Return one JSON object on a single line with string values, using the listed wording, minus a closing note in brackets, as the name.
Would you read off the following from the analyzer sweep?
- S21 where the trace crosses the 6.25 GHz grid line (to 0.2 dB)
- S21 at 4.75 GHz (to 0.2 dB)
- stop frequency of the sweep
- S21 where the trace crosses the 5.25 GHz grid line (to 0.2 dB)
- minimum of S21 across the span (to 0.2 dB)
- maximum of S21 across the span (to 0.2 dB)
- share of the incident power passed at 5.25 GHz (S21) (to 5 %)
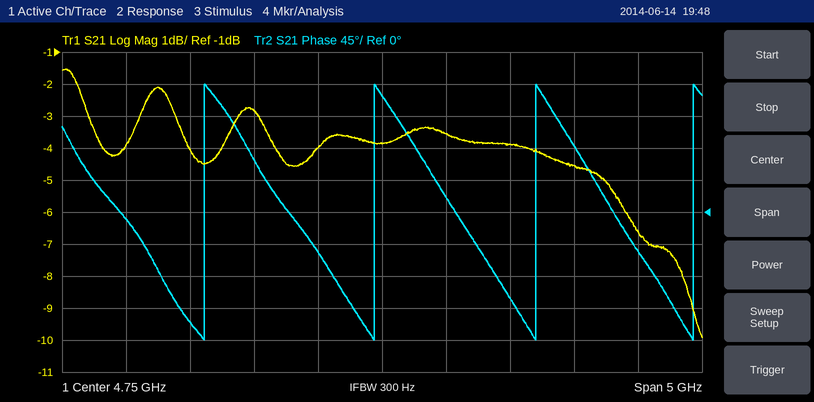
{"S21 where the trace crosses the 6.25 GHz grid line": "-4.6 dB", "S21 at 4.75 GHz": "-3.8 dB", "stop frequency of the sweep": "7.25 GHz", "S21 where the trace crosses the 5.25 GHz grid line": "-3.6 dB", "minimum of S21 across the span": "-10.0 dB", "maximum of S21 across the span": "-1.6 dB", "share of the incident power passed at 5.25 GHz (S21)": "45 %"}
